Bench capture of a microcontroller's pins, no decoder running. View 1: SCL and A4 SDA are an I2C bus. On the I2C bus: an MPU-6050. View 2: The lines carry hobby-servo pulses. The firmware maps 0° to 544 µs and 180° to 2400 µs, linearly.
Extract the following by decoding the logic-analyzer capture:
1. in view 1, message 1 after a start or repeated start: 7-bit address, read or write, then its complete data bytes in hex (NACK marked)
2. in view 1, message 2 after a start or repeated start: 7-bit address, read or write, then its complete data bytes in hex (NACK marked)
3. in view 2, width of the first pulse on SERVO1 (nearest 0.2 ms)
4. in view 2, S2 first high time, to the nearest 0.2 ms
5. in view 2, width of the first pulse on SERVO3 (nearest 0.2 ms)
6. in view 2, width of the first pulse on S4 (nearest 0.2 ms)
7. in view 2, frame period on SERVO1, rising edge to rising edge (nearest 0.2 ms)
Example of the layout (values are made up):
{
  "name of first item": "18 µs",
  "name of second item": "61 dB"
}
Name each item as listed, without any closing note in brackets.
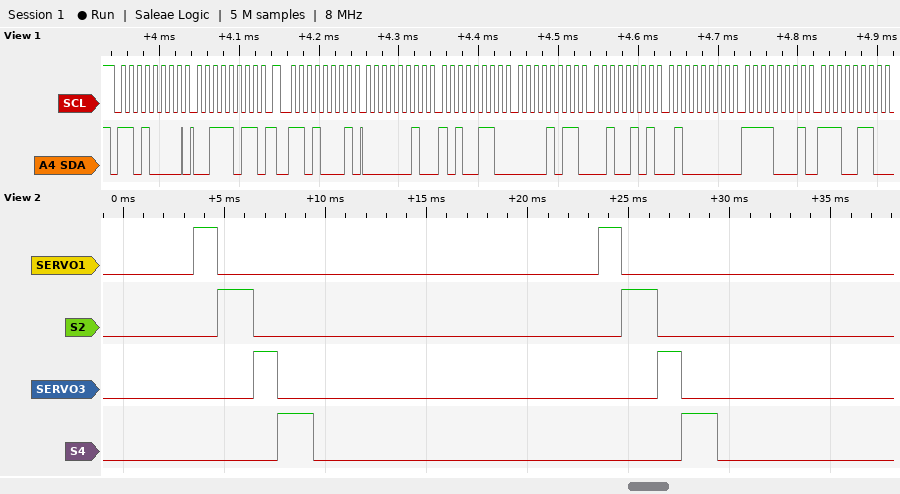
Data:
{
  "in view 1, message 1 after a start or repeated start: 7-bit address, read or write, then its complete data bytes in hex": "0x68 write: 3B",
  "in view 1, message 2 after a start or repeated start: 7-bit address, read or write, then its complete data bytes in hex": "0x68 read: 02 A6 0B 25 40 F1 E6",
  "in view 2, width of the first pulse on SERVO1": "1.2 ms",
  "in view 2, S2 first high time, to the nearest 0.2 ms": "1.8 ms",
  "in view 2, width of the first pulse on SERVO3": "1.2 ms",
  "in view 2, width of the first pulse on S4": "1.8 ms",
  "in view 2, frame period on SERVO1, rising edge to rising edge": "20.0 ms"
}
